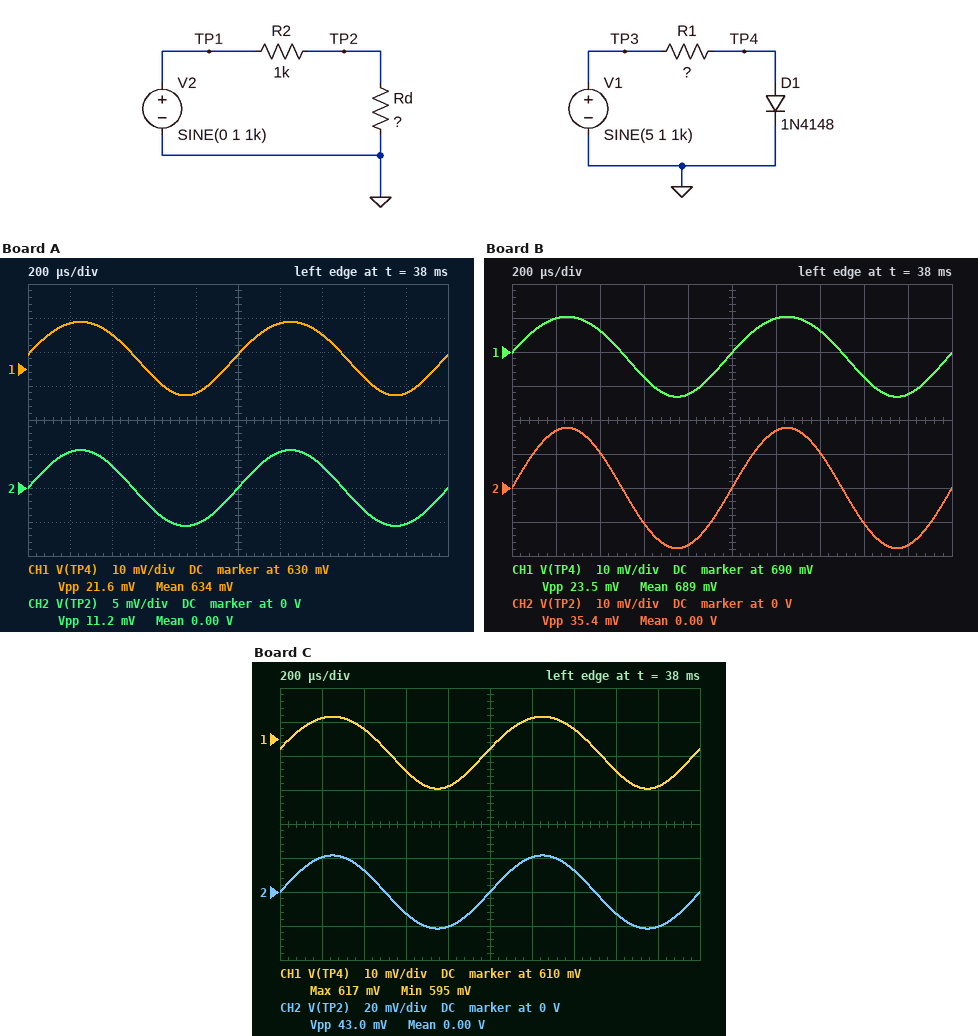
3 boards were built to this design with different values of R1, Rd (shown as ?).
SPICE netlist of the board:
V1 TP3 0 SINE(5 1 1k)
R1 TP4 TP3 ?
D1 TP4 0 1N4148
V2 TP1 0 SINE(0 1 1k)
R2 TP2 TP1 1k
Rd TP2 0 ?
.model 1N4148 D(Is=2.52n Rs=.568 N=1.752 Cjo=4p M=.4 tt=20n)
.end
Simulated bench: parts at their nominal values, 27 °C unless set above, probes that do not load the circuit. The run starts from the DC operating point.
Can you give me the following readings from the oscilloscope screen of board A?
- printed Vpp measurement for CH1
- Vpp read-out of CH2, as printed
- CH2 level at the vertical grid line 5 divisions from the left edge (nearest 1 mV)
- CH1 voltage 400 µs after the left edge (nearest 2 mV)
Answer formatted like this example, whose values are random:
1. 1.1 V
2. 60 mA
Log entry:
1. 21.6 mV
2. 11.2 mV
3. 0 V
4. 640 mV
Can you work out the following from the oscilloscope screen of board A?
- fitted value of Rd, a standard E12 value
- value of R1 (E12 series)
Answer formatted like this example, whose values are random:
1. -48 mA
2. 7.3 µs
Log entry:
1. 5.6 Ω
2. 1.5 kΩ
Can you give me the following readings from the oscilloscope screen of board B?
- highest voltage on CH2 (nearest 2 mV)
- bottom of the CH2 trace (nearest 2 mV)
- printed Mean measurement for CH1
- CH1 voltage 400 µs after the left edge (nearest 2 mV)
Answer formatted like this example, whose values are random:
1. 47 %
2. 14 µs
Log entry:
1. 18 mV
2. -18 mV
3. 689 mV
4. 696 mV
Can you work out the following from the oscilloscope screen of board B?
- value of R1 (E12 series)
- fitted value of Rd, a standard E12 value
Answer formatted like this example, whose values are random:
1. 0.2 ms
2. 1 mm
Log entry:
1. 470 Ω
2. 18 Ω
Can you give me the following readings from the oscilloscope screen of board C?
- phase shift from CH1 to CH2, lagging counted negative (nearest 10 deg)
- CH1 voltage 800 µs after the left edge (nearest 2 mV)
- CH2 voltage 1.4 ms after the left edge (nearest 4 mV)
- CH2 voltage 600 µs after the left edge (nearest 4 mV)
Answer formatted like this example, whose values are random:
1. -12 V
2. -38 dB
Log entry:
1. 0 deg
2. 596 mV
3. 12 mV
4. -12 mV
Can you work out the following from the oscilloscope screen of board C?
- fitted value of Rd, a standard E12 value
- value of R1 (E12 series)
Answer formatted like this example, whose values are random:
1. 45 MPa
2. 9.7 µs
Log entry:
1. 22 Ω
2. 2.7 kΩ
